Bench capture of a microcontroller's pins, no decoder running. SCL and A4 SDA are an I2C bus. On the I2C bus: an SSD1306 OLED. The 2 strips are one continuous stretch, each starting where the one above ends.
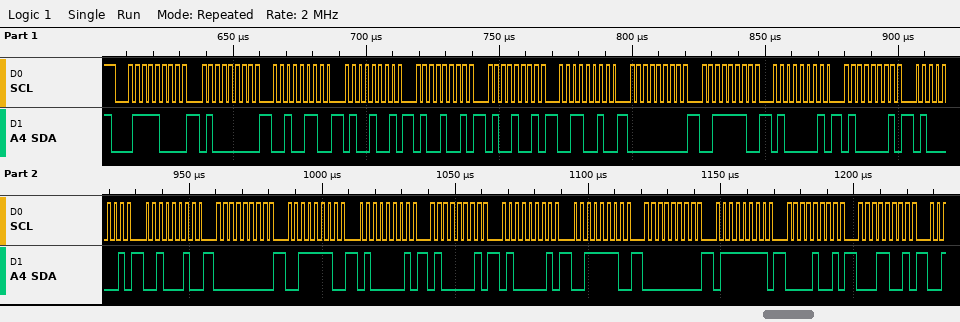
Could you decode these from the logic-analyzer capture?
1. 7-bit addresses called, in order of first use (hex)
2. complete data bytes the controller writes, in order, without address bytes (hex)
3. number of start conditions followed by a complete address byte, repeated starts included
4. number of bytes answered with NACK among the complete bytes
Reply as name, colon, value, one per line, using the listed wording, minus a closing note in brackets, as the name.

7-bit addresses called, in order of first use: 0x3C
complete data bytes the controller writes, in order, without address bytes: 40 26 49 49 49 32 00 3E 41 41 41 22 00 3E 41 41 41 3E 00 7F 09 19
number of start conditions followed by a complete address byte, repeated starts included: 1
number of bytes answered with NACK among the complete bytes: 0
